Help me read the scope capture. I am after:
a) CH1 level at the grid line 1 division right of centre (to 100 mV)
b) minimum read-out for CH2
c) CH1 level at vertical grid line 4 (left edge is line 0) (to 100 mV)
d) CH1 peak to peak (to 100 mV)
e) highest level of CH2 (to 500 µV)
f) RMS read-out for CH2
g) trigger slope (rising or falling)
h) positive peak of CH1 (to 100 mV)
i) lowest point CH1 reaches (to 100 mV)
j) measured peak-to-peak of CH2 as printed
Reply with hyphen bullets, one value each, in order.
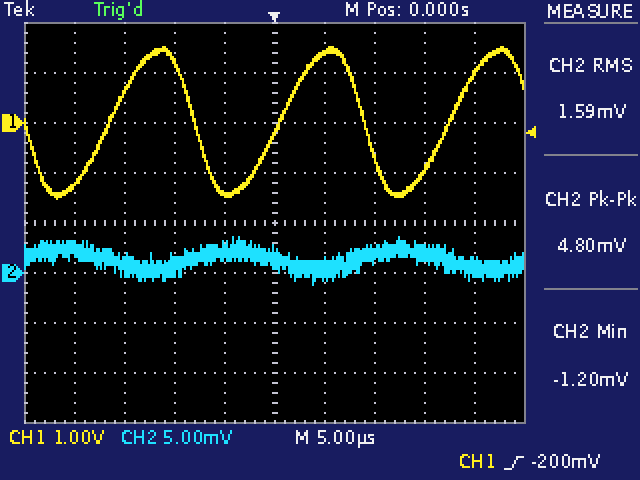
- 1.4 V
- -1.20 mV
- -1.4 V
- 3.0 V
- 3.5 mV
- 1.59 mV
- rising
- 1.5 V
- -1.5 V
- 4.80 mV
